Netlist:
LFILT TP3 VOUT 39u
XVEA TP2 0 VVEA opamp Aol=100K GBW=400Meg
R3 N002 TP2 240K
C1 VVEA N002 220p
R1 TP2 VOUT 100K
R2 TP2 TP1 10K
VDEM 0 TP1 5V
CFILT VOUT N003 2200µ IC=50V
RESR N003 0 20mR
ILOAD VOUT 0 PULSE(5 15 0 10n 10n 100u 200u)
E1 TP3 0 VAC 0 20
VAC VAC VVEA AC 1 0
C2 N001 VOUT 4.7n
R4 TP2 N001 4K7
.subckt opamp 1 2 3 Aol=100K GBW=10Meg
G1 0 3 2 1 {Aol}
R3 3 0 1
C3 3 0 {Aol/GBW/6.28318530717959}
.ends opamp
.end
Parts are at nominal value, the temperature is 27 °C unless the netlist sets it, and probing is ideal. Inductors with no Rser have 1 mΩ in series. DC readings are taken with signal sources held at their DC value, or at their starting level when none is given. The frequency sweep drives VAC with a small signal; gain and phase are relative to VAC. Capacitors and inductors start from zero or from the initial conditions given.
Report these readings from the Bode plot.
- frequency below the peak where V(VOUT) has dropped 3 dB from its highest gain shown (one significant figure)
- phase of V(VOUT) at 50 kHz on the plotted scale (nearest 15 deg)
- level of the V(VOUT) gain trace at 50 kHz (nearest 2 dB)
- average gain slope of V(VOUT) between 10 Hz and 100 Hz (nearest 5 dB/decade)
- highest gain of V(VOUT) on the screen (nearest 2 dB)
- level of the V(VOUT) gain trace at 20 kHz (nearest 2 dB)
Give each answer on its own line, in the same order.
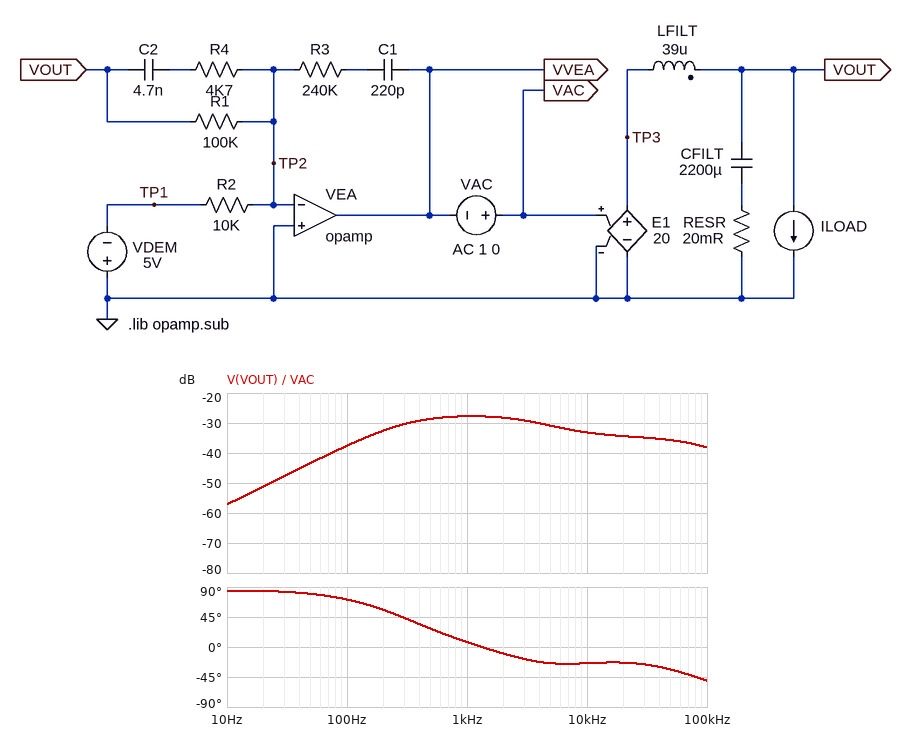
300 Hz
-30 deg
-36 dB
20 dB/decade
-28 dB
-34 dB
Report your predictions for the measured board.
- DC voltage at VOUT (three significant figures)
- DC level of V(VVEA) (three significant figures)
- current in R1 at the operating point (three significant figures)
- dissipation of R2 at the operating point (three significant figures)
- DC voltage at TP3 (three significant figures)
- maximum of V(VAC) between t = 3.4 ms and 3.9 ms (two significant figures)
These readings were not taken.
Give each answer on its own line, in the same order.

50.0 V
2.50 V
500 µA
2.50 mW
50.0 V
13 V
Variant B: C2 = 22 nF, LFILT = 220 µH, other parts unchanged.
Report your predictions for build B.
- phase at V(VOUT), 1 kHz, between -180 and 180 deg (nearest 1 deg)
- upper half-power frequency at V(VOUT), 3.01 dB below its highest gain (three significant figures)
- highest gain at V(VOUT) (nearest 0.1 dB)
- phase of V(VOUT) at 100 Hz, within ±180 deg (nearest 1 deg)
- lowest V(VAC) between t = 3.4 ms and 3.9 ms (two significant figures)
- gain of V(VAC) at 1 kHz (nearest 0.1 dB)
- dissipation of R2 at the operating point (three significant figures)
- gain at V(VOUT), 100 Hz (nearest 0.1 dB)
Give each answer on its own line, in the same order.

19 deg
16.8 kHz
-33.3 dB
36 deg
-8.8 V
-40.4 dB
2.50 mW
-42.1 dB
